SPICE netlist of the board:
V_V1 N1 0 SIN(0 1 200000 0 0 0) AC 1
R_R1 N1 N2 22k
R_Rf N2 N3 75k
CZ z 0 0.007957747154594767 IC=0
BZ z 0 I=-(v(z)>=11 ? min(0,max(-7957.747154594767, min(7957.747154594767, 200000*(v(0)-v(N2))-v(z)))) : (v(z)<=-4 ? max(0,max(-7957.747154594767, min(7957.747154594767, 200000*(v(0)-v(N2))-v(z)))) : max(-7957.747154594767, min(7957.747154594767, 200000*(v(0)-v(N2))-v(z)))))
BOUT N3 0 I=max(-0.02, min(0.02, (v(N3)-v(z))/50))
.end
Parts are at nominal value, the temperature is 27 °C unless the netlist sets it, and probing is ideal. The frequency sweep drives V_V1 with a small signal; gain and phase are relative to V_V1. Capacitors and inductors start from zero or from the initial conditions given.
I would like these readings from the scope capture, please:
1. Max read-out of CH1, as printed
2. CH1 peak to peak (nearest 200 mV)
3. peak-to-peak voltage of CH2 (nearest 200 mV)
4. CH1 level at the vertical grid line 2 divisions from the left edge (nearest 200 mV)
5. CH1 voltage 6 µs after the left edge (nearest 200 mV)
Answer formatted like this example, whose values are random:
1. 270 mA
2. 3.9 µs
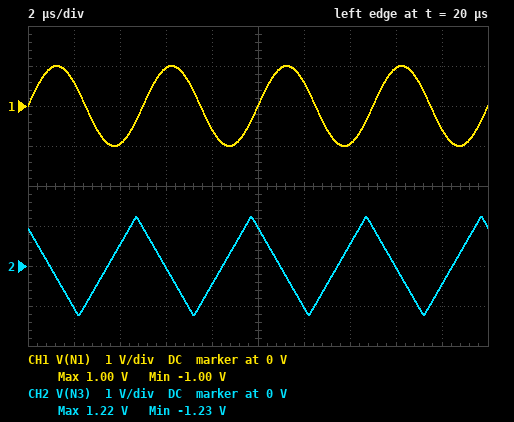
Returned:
1. 1.00 V
2. 2.0 V
3. 2.4 V
4. -1.0 V
5. 1.0 V
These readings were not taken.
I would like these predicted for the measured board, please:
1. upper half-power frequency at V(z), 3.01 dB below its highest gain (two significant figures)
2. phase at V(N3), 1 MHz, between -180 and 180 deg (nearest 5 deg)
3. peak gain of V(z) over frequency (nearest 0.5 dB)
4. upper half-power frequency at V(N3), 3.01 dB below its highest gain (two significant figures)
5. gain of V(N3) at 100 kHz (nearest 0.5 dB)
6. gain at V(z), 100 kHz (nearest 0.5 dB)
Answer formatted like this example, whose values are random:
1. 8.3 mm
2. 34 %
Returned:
1. 910 kHz
2. 130 deg
3. 10.5 dB
4. 910 kHz
5. 10.5 dB
6. 10.5 dB
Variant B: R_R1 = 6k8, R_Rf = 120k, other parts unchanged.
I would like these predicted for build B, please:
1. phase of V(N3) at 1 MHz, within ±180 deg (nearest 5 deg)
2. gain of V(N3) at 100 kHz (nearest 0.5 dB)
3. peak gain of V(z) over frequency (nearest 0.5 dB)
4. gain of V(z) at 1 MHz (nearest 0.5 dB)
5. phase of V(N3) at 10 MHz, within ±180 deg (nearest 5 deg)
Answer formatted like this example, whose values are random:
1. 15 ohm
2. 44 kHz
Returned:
1. 100 deg
2. 24.0 dB
3. 25.0 dB
4. 11.5 dB
5. 90 deg
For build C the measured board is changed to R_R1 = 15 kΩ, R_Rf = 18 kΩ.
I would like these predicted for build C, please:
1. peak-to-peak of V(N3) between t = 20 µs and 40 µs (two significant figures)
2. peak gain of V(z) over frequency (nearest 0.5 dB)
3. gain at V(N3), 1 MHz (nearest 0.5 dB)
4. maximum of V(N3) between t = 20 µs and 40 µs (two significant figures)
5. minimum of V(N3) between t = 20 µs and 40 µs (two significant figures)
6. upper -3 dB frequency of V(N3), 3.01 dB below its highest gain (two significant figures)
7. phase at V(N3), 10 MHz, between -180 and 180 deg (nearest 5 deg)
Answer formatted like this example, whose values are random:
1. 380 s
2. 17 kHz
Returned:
1. 2.3 V
2. 1.5 dB
3. 0.5 dB
4. 1.1 V
5. -1.1 V
6. 1.8 MHz
7. 100 deg
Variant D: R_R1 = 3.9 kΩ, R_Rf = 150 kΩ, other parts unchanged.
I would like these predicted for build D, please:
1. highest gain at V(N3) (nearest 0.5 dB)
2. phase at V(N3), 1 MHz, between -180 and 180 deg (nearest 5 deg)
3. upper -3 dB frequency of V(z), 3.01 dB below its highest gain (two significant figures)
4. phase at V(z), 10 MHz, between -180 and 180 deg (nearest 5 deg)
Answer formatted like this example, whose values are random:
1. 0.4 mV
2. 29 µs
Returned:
1. 31.5 dB
2. 95 deg
3. 100 kHz
4. 90 deg
